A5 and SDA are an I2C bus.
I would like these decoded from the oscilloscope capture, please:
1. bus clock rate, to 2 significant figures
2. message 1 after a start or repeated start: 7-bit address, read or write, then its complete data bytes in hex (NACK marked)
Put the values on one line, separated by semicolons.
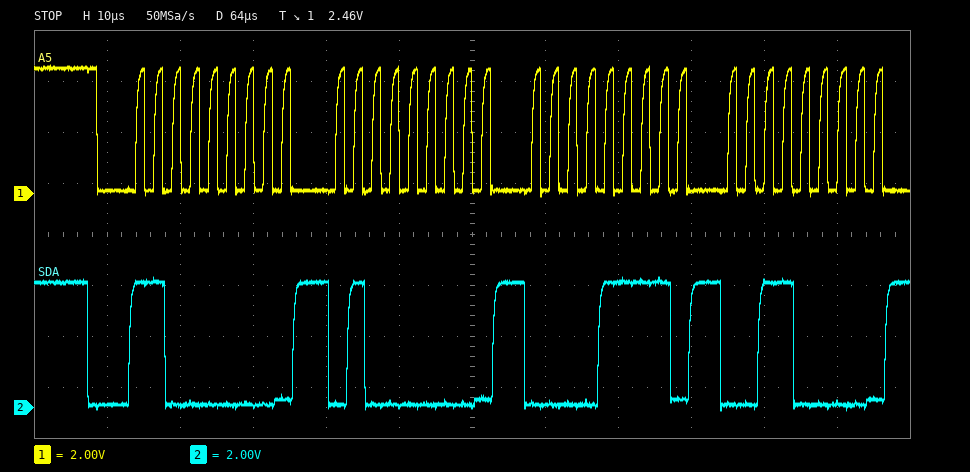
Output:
400 kHz; 0x60 write: 40 0F 30
